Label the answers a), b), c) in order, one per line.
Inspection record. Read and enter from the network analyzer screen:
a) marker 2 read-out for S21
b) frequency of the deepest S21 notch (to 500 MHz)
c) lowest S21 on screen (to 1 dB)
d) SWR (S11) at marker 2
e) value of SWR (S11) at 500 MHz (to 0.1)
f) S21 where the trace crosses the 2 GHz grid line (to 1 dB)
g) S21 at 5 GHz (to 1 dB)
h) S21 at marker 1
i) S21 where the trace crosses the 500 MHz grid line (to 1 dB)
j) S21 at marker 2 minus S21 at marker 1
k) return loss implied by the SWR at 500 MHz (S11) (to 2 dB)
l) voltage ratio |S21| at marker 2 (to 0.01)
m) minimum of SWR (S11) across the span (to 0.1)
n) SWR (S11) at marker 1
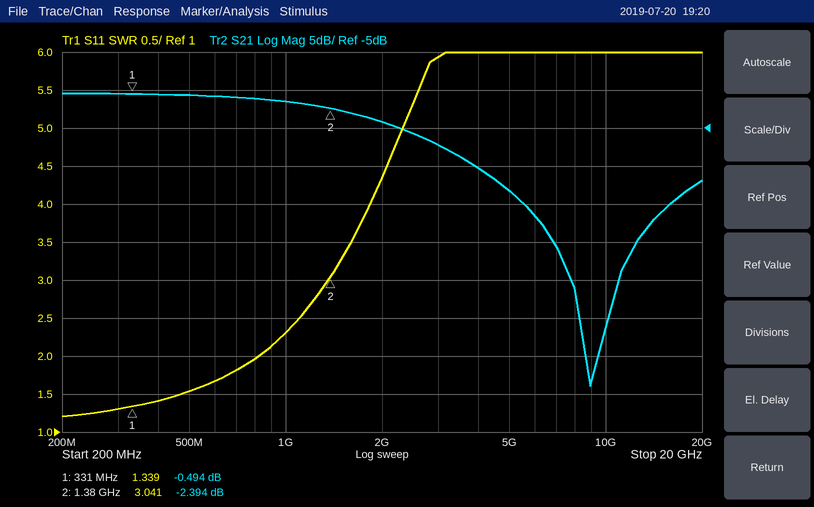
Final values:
a) -2.394 dB
b) 9.0 GHz
c) -39 dB
d) 3.041
e) 1.5
f) -4 dB
g) -13 dB
h) -0.494 dB
i) -1 dB
j) -1.900 dB
k) 14 dB
l) 0.76
m) 1.2
n) 1.339
